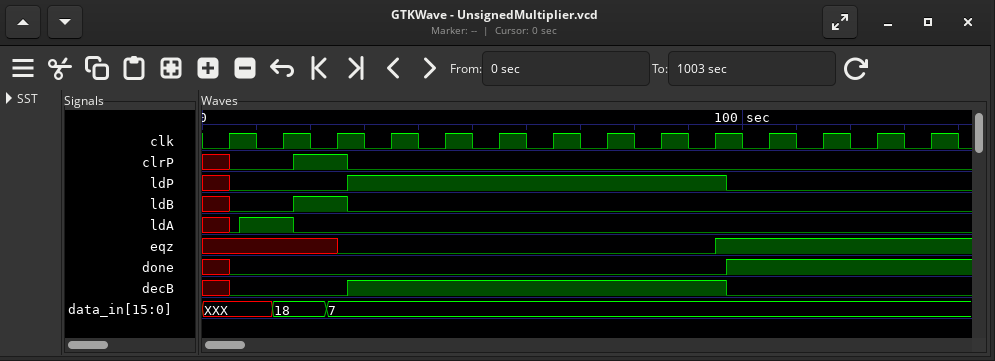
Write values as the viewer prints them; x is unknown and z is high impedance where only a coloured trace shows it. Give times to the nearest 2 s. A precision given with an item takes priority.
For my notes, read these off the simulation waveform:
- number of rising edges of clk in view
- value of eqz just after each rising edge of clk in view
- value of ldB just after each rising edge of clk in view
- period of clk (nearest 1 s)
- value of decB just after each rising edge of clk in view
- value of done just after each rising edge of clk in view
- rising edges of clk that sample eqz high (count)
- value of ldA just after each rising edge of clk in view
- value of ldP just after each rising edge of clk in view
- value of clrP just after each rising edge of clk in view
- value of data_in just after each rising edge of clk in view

14
x x 0 0 0 0 0 0 0 1 1 1 1 1
0 0 1 0 0 0 0 0 0 0 0 0 0 0
10 s
0 0 0 1 1 1 1 1 1 1 0 0 0 0
0 0 0 0 0 0 0 0 0 0 1 1 1 1
4
0 1 0 0 0 0 0 0 0 0 0 0 0 0
0 0 0 1 1 1 1 1 1 1 0 0 0 0
0 0 1 0 0 0 0 0 0 0 0 0 0 0
XXX, 18, 7, 7, 7, 7, 7, 7, 7, 7, 7, 7, 7, 7
